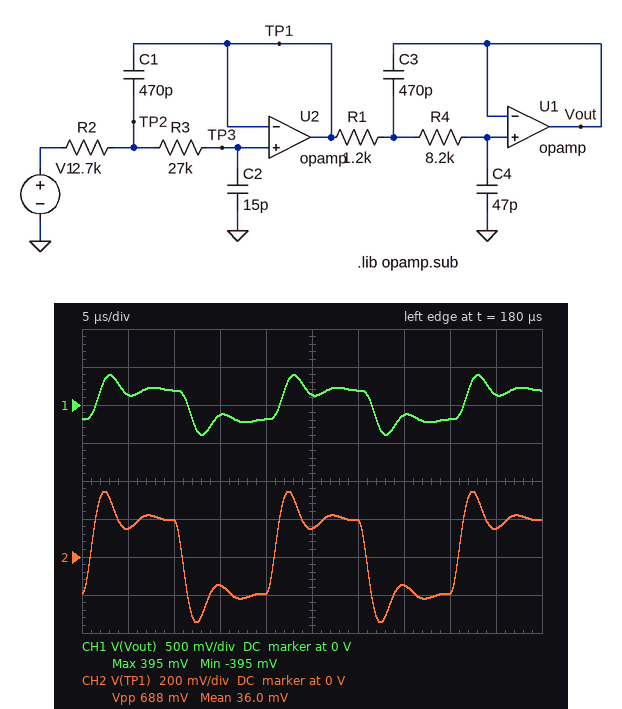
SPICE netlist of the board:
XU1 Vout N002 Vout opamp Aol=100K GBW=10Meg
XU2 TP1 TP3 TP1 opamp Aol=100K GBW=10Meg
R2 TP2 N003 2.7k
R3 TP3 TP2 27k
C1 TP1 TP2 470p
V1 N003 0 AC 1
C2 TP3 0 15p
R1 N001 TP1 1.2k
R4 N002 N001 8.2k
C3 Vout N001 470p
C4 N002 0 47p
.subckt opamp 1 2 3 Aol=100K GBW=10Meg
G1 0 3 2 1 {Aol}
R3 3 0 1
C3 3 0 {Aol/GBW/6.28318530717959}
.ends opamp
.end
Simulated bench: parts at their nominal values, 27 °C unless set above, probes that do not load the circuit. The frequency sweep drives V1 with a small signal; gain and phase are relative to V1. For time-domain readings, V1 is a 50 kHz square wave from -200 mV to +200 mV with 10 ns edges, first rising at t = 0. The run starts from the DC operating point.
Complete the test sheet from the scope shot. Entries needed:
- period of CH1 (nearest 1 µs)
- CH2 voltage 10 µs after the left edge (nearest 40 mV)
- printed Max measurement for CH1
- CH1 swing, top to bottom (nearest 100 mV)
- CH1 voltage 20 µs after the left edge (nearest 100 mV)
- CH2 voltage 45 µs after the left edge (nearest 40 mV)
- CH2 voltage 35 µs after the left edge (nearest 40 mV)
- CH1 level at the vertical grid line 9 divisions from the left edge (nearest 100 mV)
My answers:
20 µs
200 mV
395 mV
800 mV
-200 mV
160 mV
-160 mV
100 mV
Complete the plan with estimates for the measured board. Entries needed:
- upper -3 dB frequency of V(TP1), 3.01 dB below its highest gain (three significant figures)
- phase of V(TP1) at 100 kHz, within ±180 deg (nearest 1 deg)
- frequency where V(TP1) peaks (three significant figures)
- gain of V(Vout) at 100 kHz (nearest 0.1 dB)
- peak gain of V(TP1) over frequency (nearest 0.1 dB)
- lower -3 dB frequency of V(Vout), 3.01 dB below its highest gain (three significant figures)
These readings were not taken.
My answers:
257 kHz
-20 deg
196 kHz
2.0 dB
4.7 dB
126 kHz
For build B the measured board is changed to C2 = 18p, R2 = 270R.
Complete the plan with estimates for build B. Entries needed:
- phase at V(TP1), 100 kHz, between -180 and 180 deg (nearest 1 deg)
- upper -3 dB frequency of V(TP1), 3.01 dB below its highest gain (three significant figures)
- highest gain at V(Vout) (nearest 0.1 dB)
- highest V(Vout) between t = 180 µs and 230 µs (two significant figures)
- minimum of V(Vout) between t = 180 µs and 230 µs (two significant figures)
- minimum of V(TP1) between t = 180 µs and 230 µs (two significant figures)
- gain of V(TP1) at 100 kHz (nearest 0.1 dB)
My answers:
-18 deg
421 kHz
0.7 dB
260 mV
-260 mV
-200 mV
-0.2 dB
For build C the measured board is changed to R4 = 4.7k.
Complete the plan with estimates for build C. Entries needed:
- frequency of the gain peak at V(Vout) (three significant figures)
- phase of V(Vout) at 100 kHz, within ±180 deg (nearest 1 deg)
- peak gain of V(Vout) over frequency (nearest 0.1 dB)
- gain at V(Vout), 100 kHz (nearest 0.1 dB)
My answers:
203 kHz
-31 deg
6.0 dB
1.9 dB
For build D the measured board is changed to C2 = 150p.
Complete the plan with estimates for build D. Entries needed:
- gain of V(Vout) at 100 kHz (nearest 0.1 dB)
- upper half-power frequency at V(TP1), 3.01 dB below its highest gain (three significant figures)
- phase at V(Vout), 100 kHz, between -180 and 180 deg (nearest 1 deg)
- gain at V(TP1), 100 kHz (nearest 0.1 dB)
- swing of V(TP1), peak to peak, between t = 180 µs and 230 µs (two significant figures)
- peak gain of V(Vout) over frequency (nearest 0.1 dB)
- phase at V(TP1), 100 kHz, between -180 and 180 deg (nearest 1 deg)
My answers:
-9.1 dB
46.4 kHz
-128 deg
-9.5 dB
350 mV
0 dB
-111 deg
